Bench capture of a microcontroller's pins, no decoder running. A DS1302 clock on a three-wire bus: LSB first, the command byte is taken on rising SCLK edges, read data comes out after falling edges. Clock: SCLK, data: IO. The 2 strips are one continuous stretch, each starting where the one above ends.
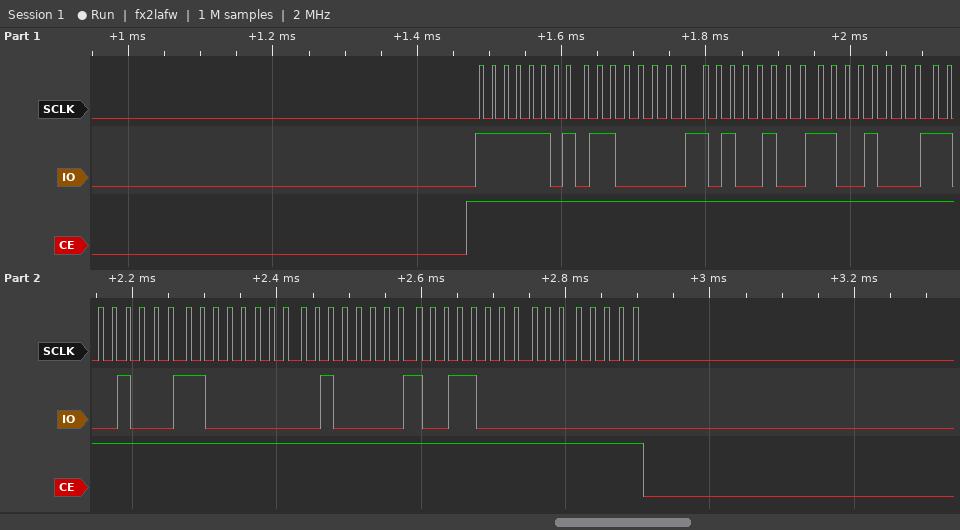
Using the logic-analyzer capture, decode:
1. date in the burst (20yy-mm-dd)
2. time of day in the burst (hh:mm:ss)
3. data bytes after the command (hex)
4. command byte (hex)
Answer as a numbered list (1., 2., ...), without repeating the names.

1. 2019-03-13
2. 13:25:06
3. 06 25 13 13 03 04 19 00
4. 0xBF
